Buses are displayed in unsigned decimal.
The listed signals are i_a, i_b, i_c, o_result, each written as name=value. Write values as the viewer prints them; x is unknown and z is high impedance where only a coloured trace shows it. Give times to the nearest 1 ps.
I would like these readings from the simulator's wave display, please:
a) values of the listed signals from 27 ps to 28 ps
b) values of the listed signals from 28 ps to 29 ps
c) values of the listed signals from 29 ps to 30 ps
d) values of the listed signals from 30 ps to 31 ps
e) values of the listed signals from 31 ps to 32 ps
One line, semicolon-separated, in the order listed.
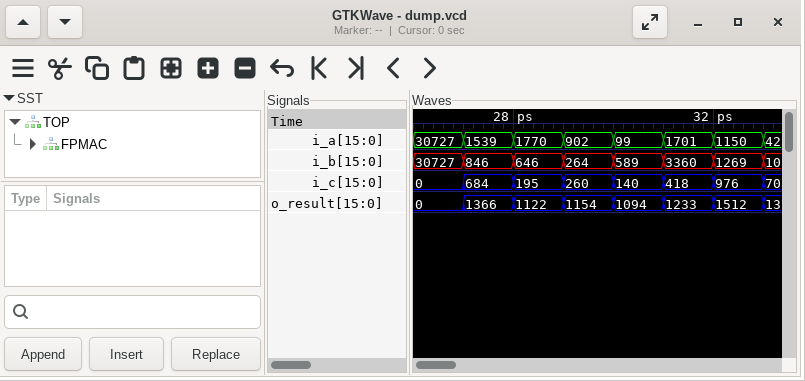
i_a=1539, i_b=846, i_c=684, o_result=1366; i_a=1770, i_b=646, i_c=195, o_result=1122; i_a=902, i_b=264, i_c=260, o_result=1154; i_a=99, i_b=589, i_c=140, o_result=1094; i_a=1701, i_b=3360, i_c=418, o_result=1233
